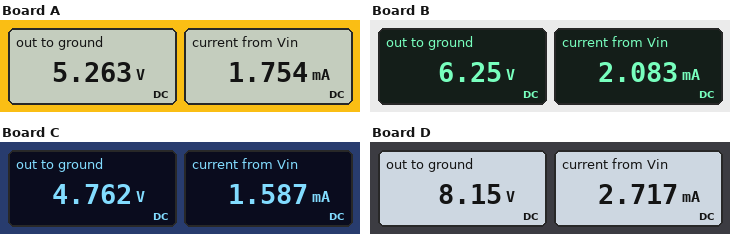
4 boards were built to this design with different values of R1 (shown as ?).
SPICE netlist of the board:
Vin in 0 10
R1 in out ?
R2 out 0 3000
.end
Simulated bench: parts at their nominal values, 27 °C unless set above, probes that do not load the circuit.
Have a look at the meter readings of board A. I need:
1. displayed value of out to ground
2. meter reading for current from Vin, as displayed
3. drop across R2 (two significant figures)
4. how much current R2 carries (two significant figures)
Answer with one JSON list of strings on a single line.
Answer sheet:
["5.263 V", "1.754 mA", "5.3 V", "1.8 mA"]
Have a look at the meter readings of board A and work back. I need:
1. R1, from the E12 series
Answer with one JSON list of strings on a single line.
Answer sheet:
["2.7 kΩ"]
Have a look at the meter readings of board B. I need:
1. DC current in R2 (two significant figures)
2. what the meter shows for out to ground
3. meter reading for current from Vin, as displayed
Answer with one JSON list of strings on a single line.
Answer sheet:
["2.1 mA", "6.25 V", "2.083 mA"]
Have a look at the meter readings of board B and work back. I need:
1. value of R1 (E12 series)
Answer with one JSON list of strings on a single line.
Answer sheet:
["1.8 kΩ"]
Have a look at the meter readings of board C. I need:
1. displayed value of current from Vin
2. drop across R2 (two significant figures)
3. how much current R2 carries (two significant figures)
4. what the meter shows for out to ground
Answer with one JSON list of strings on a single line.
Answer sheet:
["1.587 mA", "4.8 V", "1.6 mA", "4.762 V"]
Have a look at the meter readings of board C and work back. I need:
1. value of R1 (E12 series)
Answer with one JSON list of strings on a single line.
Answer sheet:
["3.3 kΩ"]
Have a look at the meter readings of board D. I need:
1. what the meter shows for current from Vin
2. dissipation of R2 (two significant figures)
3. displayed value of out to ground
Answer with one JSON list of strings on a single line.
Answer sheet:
["2.717 mA", "22 mW", "8.15 V"]
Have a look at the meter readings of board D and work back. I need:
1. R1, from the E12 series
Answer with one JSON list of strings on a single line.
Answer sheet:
["680 Ω"]
